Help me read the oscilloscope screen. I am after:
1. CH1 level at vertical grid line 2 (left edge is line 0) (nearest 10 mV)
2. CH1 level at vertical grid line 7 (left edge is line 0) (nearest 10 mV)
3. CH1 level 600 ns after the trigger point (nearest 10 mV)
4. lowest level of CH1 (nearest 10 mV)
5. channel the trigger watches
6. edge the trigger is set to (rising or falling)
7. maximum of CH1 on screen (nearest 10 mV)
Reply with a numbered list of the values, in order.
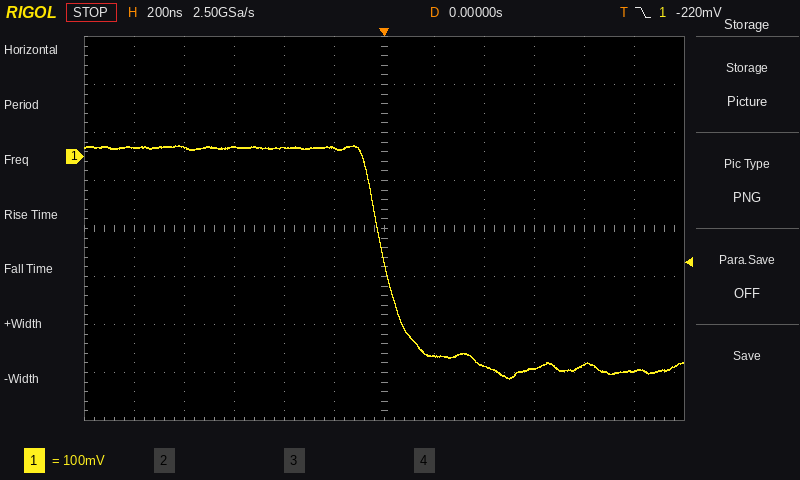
1. 20 mV
2. -420 mV
3. -440 mV
4. -460 mV
5. CH1
6. falling
7. 20 mV
